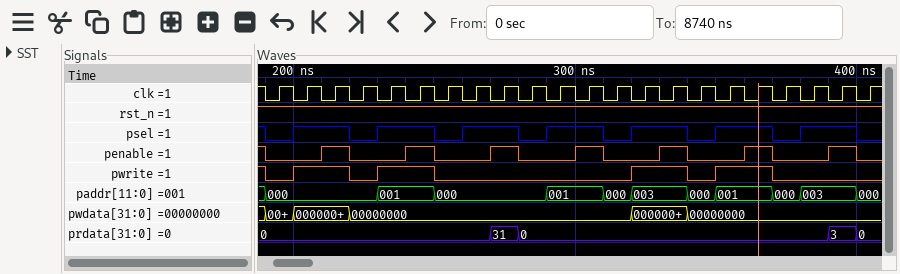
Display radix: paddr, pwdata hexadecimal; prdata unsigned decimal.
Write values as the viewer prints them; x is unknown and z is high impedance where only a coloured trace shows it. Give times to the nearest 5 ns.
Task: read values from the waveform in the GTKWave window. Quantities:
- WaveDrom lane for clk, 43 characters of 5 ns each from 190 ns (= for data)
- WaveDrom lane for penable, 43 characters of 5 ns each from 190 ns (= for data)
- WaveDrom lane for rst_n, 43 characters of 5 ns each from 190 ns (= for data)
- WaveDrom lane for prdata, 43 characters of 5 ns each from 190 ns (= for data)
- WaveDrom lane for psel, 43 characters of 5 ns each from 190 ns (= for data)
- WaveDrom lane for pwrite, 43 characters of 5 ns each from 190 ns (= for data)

{name: 'clk', wave: '0101010101010101010101010101010101010101010'}
{name: 'penable', wave: '0...1.0...1.0...1.0...1.0...1.0...1.0...1.0'}
{name: 'rst_n', wave: '1..........................................'}
{name: 'prdata', wave: '=...............=.=.....................=.=', data: '0 31 0 3 0'}
{name: 'psel', wave: '0.1...0.1...0.1...0.1...0.1...0.1...0.1...0'}
{name: 'pwrite', wave: '0.1...0.1...0.............1...0.1...0......'}
